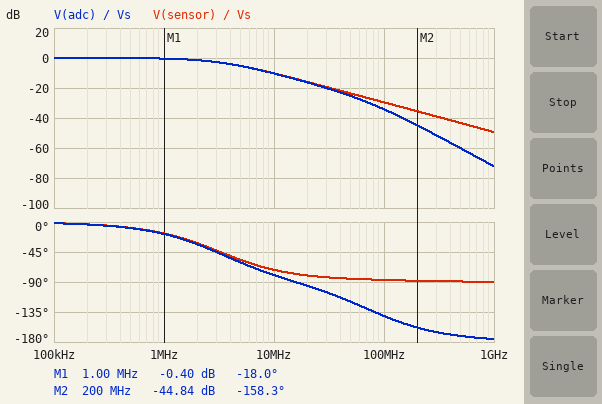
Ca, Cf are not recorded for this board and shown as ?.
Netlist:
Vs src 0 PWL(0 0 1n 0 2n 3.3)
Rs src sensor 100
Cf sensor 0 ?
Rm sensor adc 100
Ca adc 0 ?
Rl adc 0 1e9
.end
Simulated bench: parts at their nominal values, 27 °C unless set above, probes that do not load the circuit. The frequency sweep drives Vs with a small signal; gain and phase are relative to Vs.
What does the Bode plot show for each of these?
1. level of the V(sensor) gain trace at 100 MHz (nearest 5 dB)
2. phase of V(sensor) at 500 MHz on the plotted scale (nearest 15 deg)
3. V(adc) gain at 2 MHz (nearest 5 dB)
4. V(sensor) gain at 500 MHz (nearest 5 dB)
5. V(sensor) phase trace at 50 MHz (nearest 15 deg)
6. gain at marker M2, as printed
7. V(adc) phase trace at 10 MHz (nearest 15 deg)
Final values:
-30 dB
-90 deg
0 dB
-45 dB
-90 deg
-44.84 dB
-75 deg
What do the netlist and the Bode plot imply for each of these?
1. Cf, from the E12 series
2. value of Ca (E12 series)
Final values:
470 pF
22 pF
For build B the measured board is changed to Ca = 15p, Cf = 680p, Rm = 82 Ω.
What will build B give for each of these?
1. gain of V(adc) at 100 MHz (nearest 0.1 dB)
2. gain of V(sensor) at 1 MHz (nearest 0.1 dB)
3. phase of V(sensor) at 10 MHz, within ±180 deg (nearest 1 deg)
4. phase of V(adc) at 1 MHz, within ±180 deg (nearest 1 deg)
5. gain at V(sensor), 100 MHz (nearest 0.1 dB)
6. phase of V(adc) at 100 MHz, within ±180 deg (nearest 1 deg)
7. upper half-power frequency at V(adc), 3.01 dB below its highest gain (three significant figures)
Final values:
-34.8 dB
-0.8 dB
-77 deg
-24 deg
-32.7 dB
-126 deg
2.29 MHz
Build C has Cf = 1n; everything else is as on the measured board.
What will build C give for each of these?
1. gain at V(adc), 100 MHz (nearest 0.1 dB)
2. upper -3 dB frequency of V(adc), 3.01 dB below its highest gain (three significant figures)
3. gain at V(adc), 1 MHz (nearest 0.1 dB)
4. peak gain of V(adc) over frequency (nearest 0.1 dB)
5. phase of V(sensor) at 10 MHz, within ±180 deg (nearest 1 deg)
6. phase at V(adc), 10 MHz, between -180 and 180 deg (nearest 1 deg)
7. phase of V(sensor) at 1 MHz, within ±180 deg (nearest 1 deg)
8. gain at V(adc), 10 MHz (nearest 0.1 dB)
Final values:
-40.7 dB
1.56 MHz
-1.5 dB
0 dB
-81 deg
-89 deg
-33 deg
-16.3 dB
